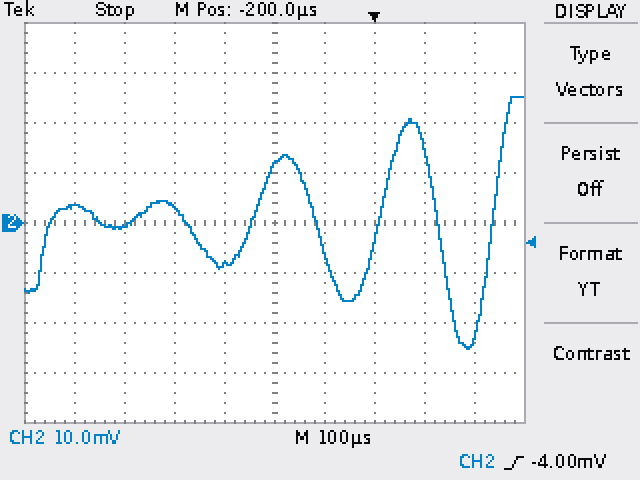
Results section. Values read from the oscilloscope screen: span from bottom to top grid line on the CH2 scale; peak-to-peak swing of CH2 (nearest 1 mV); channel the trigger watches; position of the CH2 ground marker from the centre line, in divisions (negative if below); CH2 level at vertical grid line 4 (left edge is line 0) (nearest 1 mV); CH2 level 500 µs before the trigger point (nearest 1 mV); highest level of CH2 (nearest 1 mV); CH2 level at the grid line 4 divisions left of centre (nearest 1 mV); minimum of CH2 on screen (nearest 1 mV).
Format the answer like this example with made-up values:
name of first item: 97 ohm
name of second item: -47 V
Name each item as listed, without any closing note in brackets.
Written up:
span from bottom to top grid line on the CH2 scale: 80 mV
peak-to-peak swing of CH2: 50 mV
channel the trigger watches: CH2
position of the CH2 ground marker from the centre line, in divisions: 0.0 div
CH2 level at vertical grid line 4 (left edge is line 0): -8 mV
CH2 level 500 µs before the trigger point: -1 mV
highest level of CH2: 25 mV
CH2 level at the grid line 4 divisions left of centre: 3 mV
minimum of CH2 on screen: -25 mV
